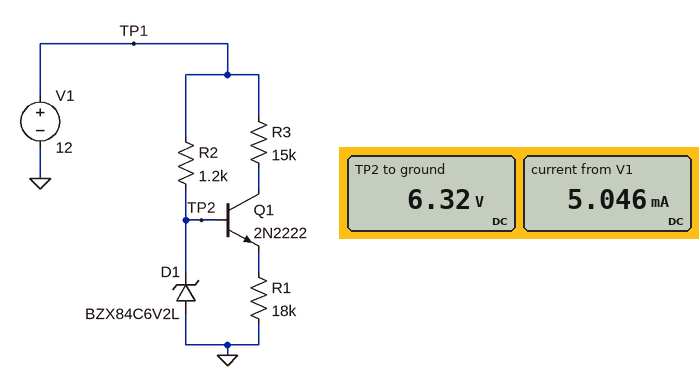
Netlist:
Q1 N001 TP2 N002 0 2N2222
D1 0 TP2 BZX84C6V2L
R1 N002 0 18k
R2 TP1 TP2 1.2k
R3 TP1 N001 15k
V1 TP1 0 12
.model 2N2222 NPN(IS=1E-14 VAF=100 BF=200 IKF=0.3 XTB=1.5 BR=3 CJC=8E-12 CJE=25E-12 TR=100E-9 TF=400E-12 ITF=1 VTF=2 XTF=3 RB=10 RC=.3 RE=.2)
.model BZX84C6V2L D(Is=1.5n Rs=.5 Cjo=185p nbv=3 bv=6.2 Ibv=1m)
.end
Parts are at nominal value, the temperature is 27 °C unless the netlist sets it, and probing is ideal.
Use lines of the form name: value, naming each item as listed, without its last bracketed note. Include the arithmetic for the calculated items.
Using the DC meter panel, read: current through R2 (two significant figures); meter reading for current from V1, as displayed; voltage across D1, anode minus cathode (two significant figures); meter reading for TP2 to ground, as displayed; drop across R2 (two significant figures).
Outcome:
current through R2: (12 V - 6.32 V) / 1.2 kΩ = 4.7 mA
meter reading for current from V1, as displayed: 5.046 mA
voltage across D1, anode minus cathode: 0 V - 6.32 V = -6.3 V
meter reading for TP2 to ground, as displayed: 6.32 V
drop across R2: 12 V - 6.32 V = 5.7 V
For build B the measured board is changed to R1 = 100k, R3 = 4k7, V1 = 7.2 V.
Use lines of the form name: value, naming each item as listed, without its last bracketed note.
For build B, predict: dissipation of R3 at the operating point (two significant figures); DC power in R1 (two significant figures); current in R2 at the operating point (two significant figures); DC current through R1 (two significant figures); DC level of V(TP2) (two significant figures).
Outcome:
dissipation of R3 at the operating point: 15 µW
DC power in R1: 310 µW
current in R2 at the operating point: 840 µA
DC current through R1: 56 µA
DC level of V(TP2): 6.2 V
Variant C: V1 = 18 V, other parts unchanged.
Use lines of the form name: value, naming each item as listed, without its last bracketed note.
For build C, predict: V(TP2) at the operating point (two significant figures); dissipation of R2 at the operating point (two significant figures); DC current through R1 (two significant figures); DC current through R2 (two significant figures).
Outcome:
V(TP2) at the operating point: 6.4 V
dissipation of R2 at the operating point: 110 mW
DC current through R1: 320 µA
DC current through R2: 9.7 mA
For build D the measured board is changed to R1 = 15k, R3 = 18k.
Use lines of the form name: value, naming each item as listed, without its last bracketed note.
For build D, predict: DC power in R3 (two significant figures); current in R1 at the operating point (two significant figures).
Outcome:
DC power in R3: 2.2 mW
current in R1 at the operating point: 380 µA
